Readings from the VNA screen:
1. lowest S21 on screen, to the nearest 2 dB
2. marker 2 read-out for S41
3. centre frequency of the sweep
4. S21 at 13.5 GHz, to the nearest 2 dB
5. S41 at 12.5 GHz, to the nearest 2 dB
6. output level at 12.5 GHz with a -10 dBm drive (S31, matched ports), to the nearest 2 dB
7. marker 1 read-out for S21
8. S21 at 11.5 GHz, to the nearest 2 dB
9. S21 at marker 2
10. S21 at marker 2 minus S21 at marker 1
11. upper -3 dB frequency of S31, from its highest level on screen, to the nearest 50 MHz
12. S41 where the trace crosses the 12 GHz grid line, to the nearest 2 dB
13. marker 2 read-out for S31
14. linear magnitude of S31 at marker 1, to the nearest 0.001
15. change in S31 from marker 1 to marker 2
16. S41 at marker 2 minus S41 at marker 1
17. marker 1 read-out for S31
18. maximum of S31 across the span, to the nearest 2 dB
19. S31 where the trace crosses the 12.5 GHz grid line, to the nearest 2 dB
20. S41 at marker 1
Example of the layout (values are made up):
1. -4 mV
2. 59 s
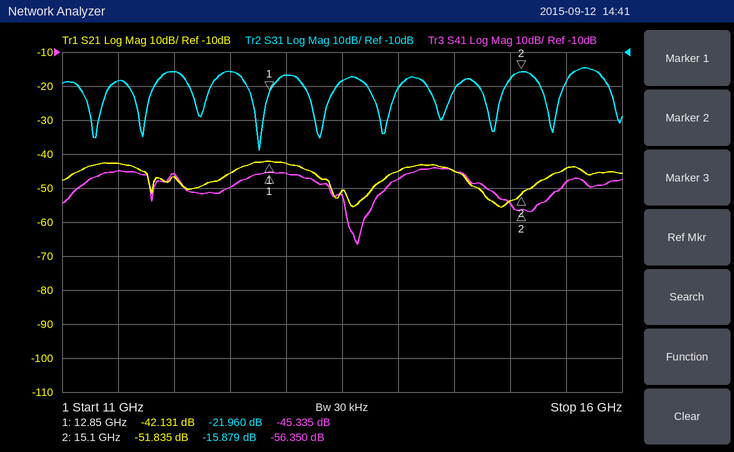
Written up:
1. -56 dB
2. -56.350 dB
3. 13.5 GHz
4. -50 dB
5. -50 dB
6. -26 dBm
7. -42.131 dB
8. -42 dB
9. -51.835 dB
10. -9.704 dB
11. 15.85 GHz
12. -46 dB
13. -15.879 dB
14. 0.080
15. 6.081 dB
16. -11.015 dB
17. -21.960 dB
18. -14 dB
19. -16 dB
20. -45.335 dB
